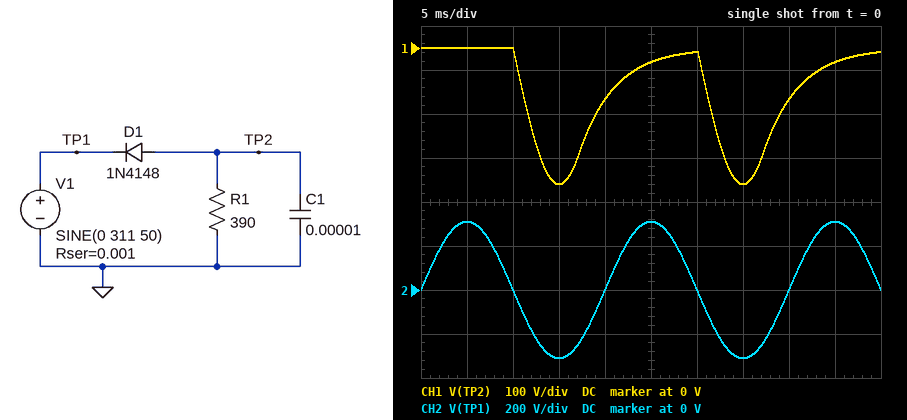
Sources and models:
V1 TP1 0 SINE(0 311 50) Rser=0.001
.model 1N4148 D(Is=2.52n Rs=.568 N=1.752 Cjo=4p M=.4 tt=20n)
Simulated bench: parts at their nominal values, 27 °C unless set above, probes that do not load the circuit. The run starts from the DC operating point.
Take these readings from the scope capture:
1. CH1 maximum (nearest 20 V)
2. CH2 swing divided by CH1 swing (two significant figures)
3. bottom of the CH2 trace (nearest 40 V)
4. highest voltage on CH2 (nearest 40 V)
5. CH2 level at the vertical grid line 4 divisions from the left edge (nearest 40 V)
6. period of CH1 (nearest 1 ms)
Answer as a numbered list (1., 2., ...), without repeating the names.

1. 0 V
2. 2.0
3. -320 V
4. 320 V
5. 0 V
6. 20 ms
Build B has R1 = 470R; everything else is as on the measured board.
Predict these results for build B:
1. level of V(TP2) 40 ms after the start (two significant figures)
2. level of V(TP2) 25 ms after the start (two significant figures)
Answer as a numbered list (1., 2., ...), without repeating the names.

1. -130 V
2. -46 V
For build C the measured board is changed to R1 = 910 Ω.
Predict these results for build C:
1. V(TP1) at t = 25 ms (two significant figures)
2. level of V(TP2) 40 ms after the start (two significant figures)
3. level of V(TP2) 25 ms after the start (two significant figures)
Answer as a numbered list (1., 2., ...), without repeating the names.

1. 310 V
2. -190 V
3. -110 V
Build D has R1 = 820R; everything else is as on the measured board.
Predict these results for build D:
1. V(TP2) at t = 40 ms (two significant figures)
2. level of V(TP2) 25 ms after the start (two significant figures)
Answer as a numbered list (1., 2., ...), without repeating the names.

1. -180 V
2. -99 V
